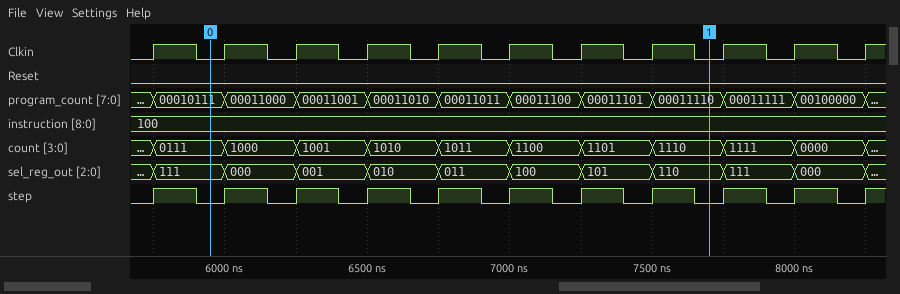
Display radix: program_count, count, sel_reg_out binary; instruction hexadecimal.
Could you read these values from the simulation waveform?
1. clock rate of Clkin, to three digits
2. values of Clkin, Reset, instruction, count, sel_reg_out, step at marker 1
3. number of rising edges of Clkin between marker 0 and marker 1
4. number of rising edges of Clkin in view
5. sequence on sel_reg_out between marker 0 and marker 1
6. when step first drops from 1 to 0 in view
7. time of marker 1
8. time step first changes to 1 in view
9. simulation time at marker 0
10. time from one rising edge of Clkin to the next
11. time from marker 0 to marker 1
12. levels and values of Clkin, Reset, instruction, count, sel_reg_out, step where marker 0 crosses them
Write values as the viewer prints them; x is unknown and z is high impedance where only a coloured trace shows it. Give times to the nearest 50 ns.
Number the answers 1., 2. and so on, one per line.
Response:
1. 4.00 MHz
2. Clkin=0, Reset=0, instruction=100, count=1110, sel_reg_out=110, step=0
3. 7
4. 11
5. 111, 000, 001, 010, 011, 100, 101, 110
6. 5900 ns
7. 7700 ns
8. 5750 ns
9. 5950 ns
10. 250 ns
11. 1750 ns
12. Clkin=0, Reset=0, instruction=100, count=0111, sel_reg_out=111, step=0
